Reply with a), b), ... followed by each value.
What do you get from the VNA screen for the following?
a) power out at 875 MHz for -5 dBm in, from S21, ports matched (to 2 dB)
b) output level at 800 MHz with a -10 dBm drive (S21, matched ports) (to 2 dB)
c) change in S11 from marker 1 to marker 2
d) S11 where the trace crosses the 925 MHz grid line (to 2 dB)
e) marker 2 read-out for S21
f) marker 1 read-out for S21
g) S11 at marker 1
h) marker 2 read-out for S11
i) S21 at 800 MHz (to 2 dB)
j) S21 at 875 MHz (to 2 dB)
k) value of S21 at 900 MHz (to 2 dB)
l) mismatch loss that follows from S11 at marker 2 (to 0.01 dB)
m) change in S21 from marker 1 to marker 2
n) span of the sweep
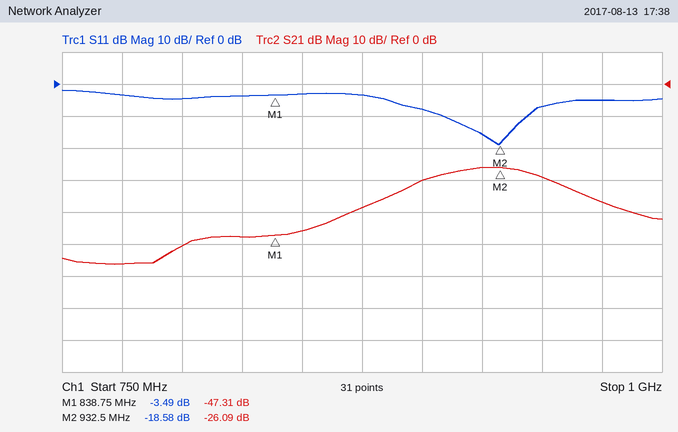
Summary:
a) -44 dBm
b) -60 dBm
c) -15.09 dB
d) -16 dB
e) -26.09 dB
f) -47.31 dB
g) -3.49 dB
h) -18.58 dB
i) -50 dB
j) -38 dB
k) -30 dB
l) 0.06 dB
m) 21.22 dB
n) 250 MHz
